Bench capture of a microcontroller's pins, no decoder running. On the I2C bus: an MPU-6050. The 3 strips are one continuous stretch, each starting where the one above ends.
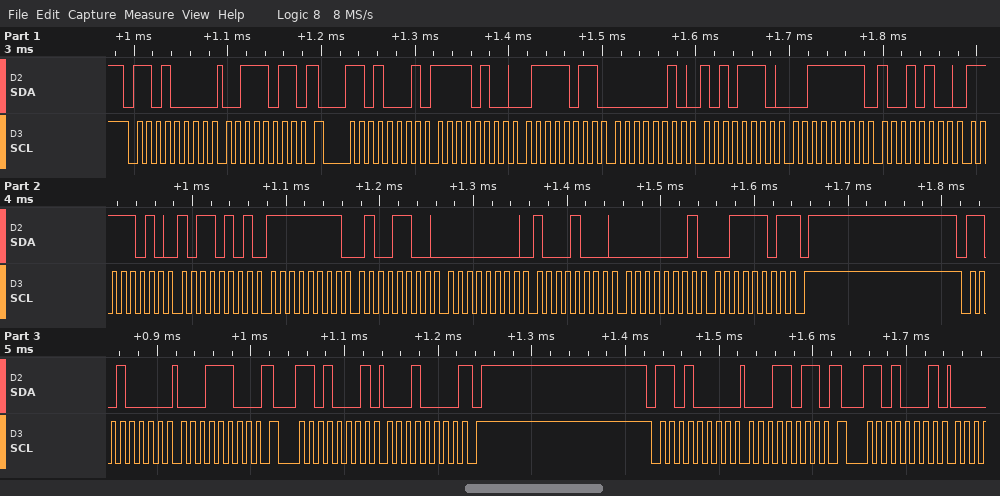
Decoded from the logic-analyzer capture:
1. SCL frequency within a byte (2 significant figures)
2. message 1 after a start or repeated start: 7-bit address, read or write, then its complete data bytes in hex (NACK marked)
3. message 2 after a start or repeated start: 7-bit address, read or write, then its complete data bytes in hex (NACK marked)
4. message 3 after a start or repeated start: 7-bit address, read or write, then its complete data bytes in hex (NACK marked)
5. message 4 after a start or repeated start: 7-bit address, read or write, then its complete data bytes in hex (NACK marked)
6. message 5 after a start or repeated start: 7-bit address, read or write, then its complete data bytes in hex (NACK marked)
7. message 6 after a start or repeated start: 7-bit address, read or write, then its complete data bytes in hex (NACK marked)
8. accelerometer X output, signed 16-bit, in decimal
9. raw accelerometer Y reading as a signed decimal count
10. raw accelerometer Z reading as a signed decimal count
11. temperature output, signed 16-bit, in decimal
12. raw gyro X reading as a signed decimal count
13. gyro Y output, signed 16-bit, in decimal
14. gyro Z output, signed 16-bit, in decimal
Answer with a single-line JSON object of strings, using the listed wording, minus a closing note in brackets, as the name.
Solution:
{"SCL frequency within a byte": "100 kHz", "message 1 after a start or repeated start: 7-bit address, read or write, then its complete data bytes in hex": "0x68 write: 3B", "message 2 after a start or repeated start: 7-bit address, read or write, then its complete data bytes in hex": "0x68 read: F4 7B 02 AE 3F 94 FA B5 FF 4C 00 88 01 3D NACK", "message 3 after a start or repeated start: 7-bit address, read or write, then its complete data bytes in hex": "0x68 write: 1C", "message 4 after a start or repeated start: 7-bit address, read or write, then its complete data bytes in hex": "0x68 read: 10 NACK", "message 5 after a start or repeated start: 7-bit address, read or write, then its complete data bytes in hex": "0x68 write: 1B", "message 6 after a start or repeated start: 7-bit address, read or write, then its complete data bytes in hex": "0x68 read", "accelerometer X output, signed 16-bit, in decimal": "-2949", "raw accelerometer Y reading as a signed decimal count": "686", "raw accelerometer Z reading as a signed decimal count": "16276", "temperature output, signed 16-bit, in decimal": "-1355", "raw gyro X reading as a signed decimal count": "-180", "gyro Y output, signed 16-bit, in decimal": "136", "gyro Z output, signed 16-bit, in decimal": "317"}
